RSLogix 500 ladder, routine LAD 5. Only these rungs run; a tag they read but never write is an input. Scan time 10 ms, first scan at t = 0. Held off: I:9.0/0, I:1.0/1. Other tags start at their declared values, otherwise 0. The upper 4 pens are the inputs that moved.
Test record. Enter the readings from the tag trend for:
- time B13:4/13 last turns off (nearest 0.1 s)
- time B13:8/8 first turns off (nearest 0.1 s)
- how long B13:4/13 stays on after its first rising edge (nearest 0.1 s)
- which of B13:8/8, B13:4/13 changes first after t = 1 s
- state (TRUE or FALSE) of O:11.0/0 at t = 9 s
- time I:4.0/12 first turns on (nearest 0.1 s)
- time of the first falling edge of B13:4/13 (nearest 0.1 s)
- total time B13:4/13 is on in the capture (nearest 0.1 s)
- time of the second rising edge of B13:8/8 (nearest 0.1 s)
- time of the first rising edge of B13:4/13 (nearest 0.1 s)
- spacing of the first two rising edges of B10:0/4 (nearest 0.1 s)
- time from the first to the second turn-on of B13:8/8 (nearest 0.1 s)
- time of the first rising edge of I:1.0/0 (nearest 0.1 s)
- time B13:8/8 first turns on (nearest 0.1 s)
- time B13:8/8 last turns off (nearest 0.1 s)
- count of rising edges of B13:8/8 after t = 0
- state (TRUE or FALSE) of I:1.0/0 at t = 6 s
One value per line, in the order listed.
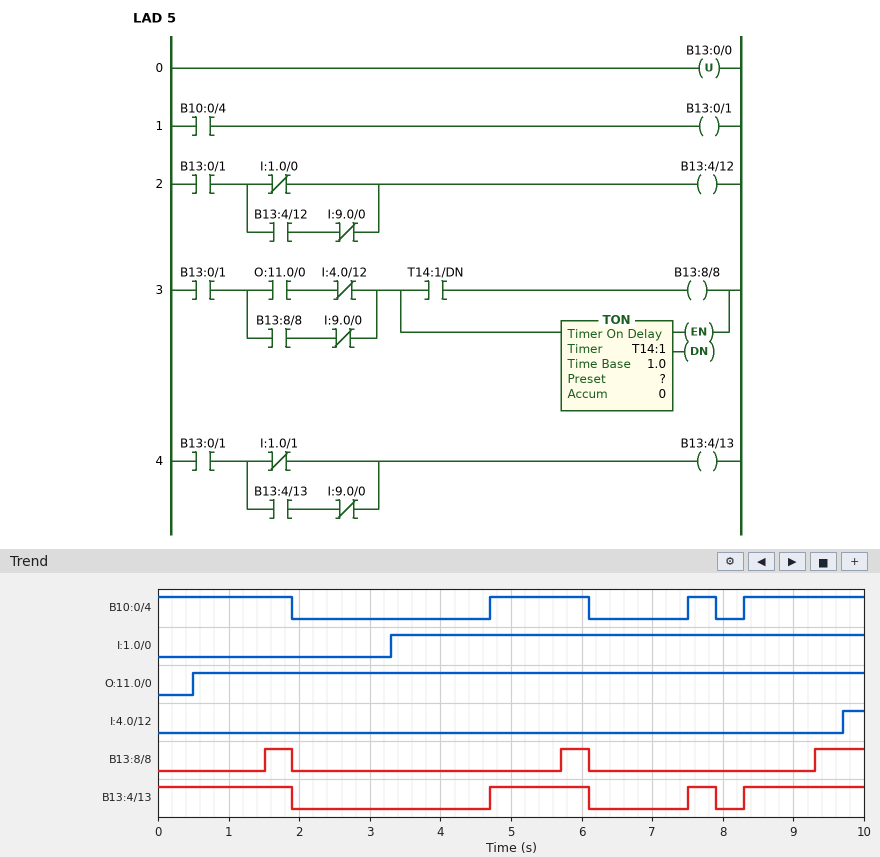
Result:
7.9 s
1.9 s
1.4 s
B13:8/8
TRUE
9.7 s
1.9 s
5.4 s
5.7 s
4.7 s
2.8 s
4.2 s
3.3 s
1.5 s
6.1 s
3
TRUE
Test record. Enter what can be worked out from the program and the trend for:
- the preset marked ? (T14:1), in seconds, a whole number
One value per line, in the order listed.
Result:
1 s
